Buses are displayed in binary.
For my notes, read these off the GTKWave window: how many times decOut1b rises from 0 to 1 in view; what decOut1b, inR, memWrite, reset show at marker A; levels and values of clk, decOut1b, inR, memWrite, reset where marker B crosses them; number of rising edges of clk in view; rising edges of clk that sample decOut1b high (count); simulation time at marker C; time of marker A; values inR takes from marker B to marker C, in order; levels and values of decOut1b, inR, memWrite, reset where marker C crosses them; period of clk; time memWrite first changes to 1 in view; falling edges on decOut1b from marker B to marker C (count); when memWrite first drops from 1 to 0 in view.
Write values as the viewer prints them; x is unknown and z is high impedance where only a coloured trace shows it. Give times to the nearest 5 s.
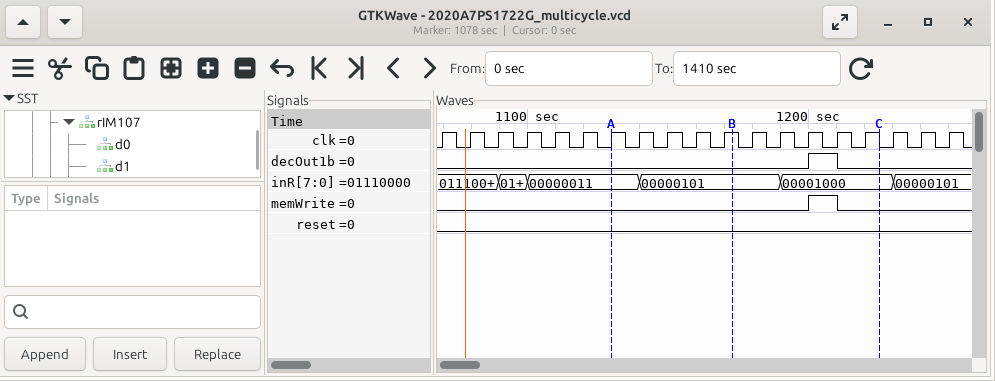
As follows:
1
decOut1b=0, inR=00000011, memWrite=0, reset=0
clk=1, decOut1b=0, inR=00000101, memWrite=0, reset=0
19
1
1225 s
1130 s
00000101, 00001000
decOut1b=0, inR=00001000, memWrite=0, reset=0
10 s
1200 s
1
1210 s
